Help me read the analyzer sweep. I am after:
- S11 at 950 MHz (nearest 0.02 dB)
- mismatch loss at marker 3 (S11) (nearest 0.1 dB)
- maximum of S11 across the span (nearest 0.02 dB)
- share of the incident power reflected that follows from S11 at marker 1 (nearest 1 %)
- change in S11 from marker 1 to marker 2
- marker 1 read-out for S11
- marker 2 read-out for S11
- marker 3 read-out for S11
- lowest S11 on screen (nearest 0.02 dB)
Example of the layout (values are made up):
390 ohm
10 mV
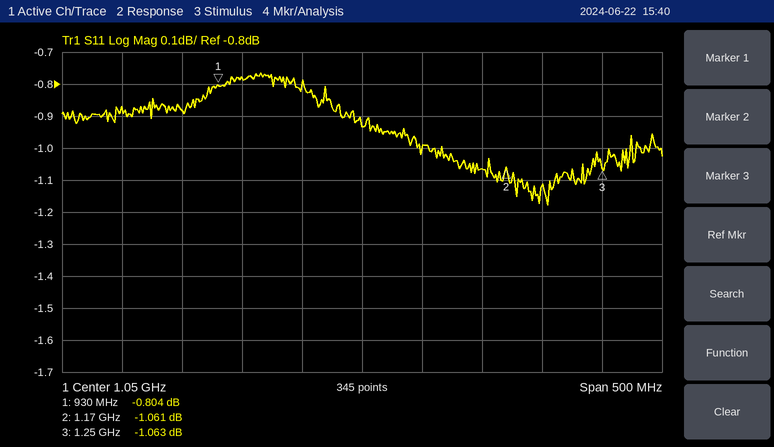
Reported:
-0.78 dB
6.6 dB
-0.76 dB
83 %
-0.257 dB
-0.804 dB
-1.061 dB
-1.063 dB
-1.18 dB
